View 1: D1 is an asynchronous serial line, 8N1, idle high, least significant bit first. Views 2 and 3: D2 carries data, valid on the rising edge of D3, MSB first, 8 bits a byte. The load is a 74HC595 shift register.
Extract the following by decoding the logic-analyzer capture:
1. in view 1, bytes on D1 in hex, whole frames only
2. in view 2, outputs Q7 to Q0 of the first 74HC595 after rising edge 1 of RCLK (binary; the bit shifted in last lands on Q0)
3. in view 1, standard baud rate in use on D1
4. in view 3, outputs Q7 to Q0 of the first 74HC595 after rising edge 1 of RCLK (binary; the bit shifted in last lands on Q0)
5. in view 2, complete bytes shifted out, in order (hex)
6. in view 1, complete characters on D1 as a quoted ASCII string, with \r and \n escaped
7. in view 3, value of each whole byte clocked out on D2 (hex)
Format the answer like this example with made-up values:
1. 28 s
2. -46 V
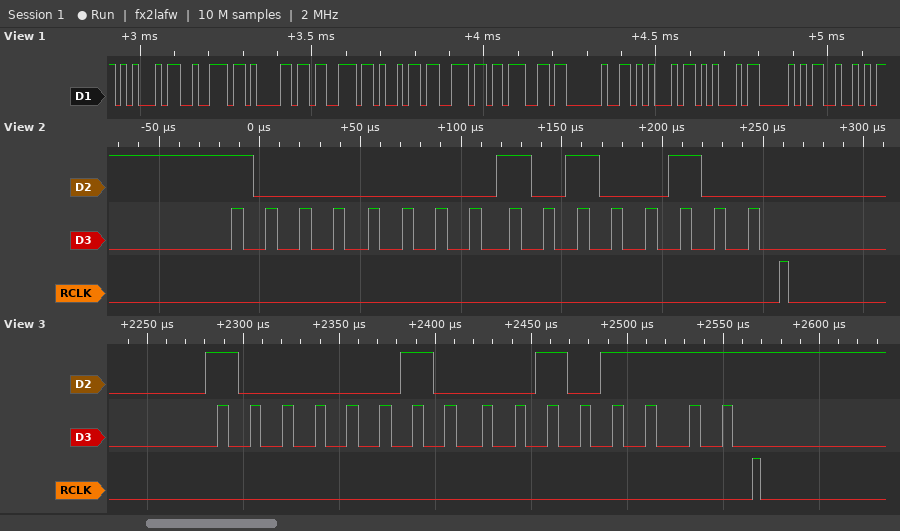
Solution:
1. 45 72 61 73 69 6E 67 20 45 45 50 52
2. 10100100
3. 57600 baud
4. 00101111
5. 80 A4
6. "Erasing EEPR"
7. 82 2F
